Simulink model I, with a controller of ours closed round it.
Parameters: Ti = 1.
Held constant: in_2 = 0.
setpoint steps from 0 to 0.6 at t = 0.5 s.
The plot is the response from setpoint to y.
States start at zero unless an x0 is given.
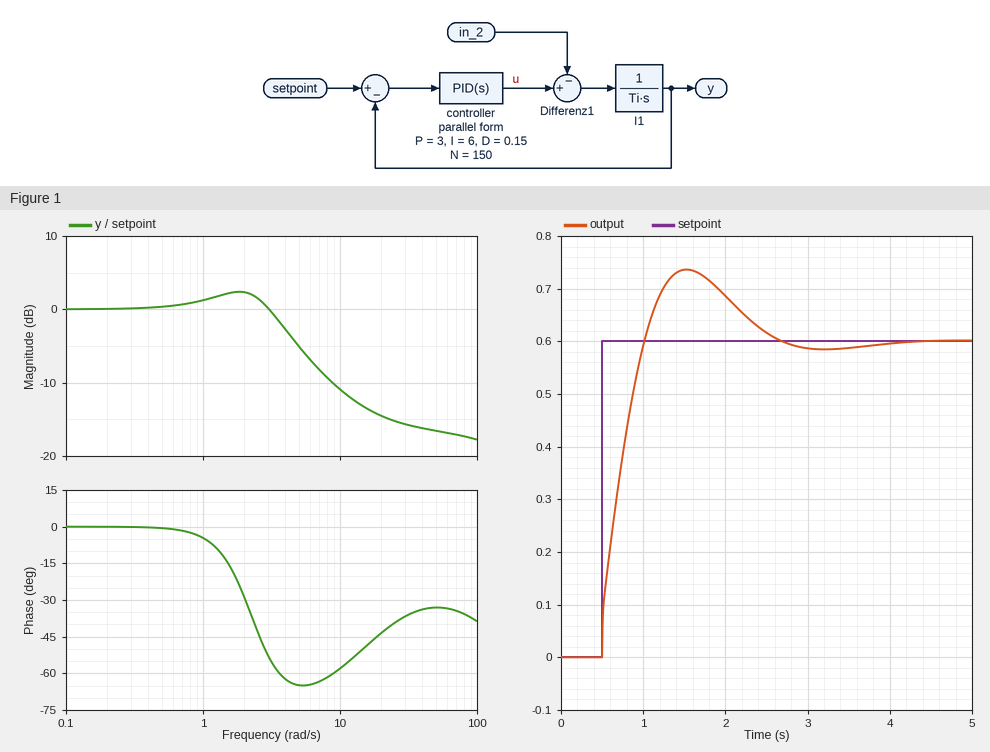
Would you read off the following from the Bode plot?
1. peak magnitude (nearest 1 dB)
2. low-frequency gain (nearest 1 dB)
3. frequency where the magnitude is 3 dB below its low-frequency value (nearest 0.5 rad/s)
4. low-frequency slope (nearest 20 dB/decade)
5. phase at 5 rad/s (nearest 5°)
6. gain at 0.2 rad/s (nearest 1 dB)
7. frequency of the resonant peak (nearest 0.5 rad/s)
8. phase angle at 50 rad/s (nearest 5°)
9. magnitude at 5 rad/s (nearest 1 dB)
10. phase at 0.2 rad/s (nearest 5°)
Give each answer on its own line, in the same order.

2 dB
0 dB
4.0 rad/s
0 dB/decade
-65°
0 dB
2.0 rad/s
-35°
-5 dB
0°
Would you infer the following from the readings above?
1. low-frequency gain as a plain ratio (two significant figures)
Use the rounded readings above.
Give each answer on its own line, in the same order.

1.0
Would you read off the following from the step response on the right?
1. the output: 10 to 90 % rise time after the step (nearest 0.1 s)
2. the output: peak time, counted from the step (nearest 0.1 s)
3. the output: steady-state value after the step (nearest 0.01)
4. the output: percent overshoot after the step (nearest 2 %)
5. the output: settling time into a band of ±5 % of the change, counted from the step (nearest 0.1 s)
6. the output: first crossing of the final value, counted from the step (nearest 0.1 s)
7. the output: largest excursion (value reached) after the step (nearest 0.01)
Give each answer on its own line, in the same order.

0.4 s
1.0 s
0.60
22 %
1.9 s
0.5 s
0.74
